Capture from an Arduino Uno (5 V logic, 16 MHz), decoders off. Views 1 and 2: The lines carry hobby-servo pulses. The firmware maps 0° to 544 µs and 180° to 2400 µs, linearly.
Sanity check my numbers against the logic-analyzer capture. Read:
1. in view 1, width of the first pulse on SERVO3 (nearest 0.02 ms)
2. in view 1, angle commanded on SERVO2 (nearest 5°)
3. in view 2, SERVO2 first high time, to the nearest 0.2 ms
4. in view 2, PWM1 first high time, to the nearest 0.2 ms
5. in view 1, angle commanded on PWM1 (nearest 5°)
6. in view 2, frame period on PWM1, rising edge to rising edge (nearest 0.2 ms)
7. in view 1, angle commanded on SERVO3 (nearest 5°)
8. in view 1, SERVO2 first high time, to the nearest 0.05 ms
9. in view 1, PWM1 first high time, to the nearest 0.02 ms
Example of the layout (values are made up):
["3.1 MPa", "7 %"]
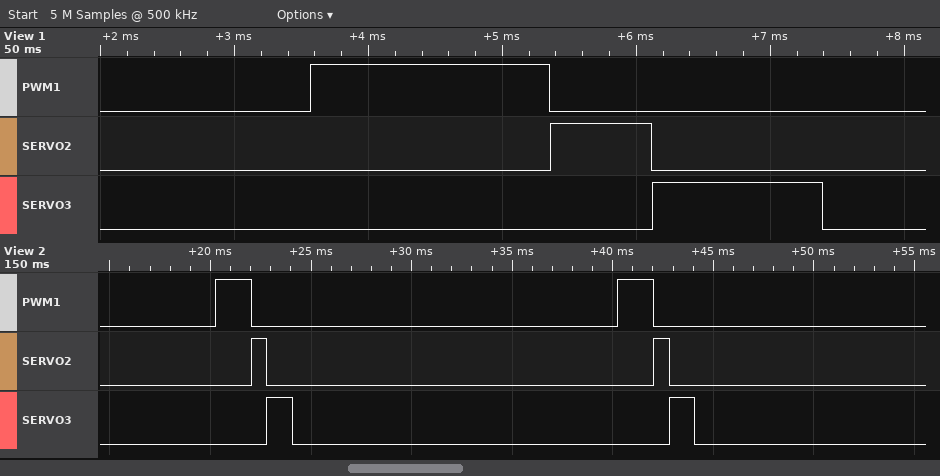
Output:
["1.26 ms", "20°", "0.8 ms", "1.8 ms", "120°", "20.0 ms", "70°", "0.75 ms", "1.78 ms"]
